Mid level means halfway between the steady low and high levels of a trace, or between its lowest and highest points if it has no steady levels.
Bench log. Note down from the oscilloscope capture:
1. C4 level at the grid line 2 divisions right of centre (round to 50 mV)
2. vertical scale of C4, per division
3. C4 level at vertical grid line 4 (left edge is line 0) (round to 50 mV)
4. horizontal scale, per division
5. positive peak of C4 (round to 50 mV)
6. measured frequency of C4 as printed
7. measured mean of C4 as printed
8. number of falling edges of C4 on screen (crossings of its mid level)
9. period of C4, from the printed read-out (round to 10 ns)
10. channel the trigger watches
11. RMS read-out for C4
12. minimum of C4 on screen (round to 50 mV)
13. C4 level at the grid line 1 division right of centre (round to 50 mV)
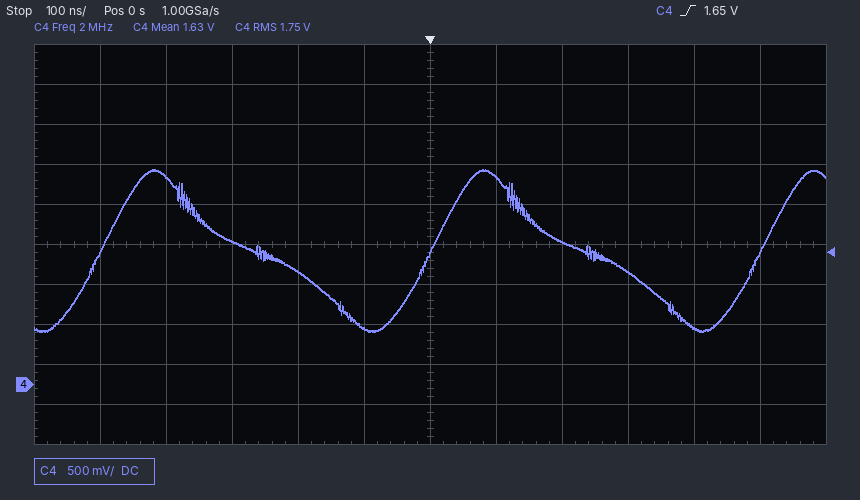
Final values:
1.80 V
500 mV
1.40 V
100 ns
2.70 V
2 MHz
1.63 V
2
500 ns
C4
1.75 V
650 mV
2.60 V
